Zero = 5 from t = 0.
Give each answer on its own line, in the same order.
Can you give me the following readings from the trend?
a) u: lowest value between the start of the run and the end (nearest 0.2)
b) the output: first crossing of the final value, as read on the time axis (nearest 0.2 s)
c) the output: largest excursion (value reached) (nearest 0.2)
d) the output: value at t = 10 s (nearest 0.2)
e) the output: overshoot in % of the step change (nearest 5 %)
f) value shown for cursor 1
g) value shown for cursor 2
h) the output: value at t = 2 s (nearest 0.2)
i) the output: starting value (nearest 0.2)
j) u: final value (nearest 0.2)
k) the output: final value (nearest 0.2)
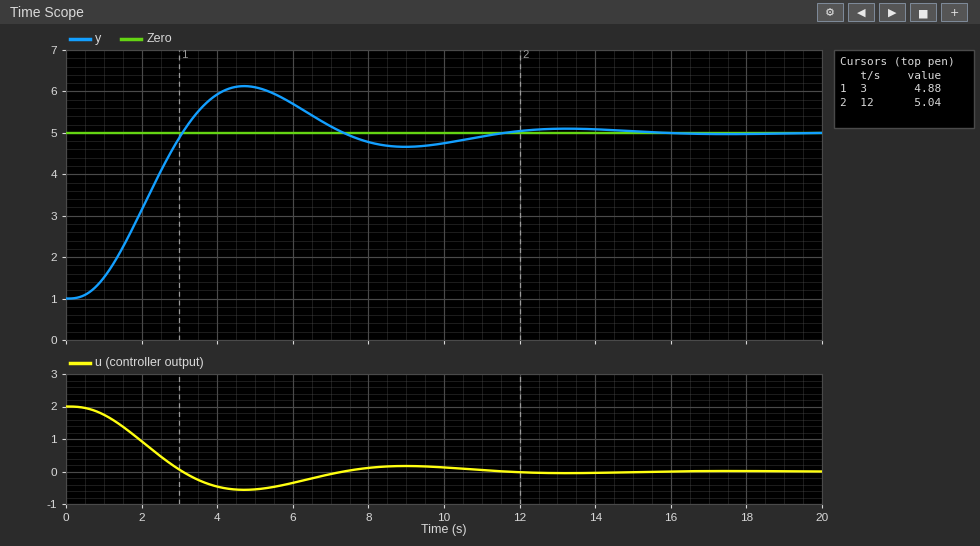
-0.6
3.0 s
6.2
4.8
30 %
4.88
5.04
3.2
1.0
0.0
5.0
